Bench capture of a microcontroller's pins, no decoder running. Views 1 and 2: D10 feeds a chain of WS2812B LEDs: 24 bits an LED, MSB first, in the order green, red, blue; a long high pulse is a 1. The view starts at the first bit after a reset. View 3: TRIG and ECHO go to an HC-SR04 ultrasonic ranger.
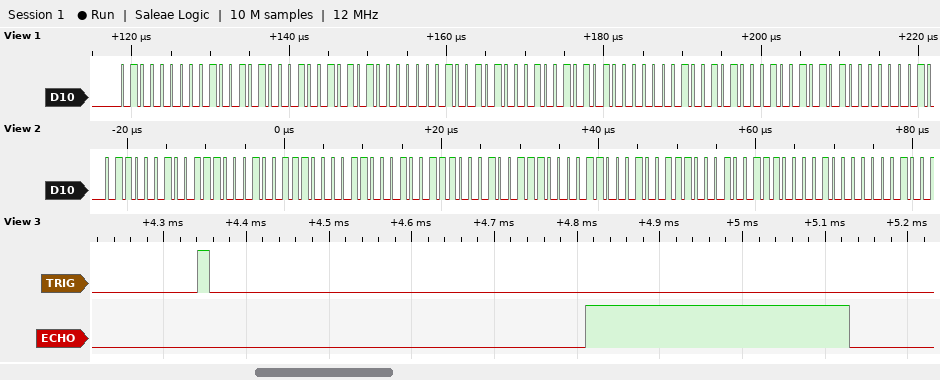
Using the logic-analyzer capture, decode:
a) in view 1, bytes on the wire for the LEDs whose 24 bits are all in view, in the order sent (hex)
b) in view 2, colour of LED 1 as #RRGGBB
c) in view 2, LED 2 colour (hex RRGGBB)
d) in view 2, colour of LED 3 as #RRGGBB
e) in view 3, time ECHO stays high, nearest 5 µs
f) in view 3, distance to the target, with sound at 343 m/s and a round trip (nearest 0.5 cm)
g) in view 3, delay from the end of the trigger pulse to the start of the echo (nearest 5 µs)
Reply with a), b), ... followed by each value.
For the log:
a) 40 4A 25 40 4A 25 40 4A 25
b) #716238
c) #716238
d) #716238
e) 320 µs
f) 5.5 cm
g) 455 µs
